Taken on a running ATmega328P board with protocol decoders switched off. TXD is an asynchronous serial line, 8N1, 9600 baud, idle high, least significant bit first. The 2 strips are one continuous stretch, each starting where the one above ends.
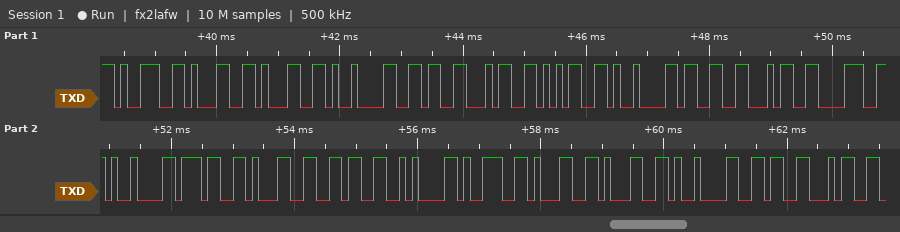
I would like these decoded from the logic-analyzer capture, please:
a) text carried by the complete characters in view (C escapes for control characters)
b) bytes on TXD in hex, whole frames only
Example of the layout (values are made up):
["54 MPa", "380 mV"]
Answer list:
["\"911\\t645\\t348\\t716\\n911\\t64\"", "39 31 31 09 36 34 35 09 33 34 38 09 37 31 36 0A 39 31 31 09 36 34"]
